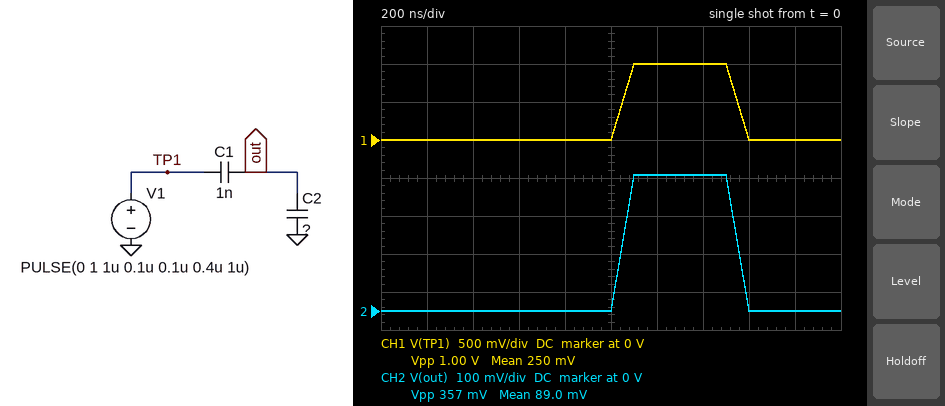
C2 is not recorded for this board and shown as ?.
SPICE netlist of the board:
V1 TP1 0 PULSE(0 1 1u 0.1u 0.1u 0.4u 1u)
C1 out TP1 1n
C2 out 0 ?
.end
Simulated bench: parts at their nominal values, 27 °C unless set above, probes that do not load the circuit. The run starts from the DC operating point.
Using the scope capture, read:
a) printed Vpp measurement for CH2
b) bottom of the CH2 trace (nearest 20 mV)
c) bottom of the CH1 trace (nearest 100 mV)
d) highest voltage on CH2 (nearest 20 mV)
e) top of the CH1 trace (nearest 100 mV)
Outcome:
357 mV
0 V
0 V
360 mV
1.0 V
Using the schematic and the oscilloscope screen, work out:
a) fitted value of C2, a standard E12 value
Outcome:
1.8 nF
